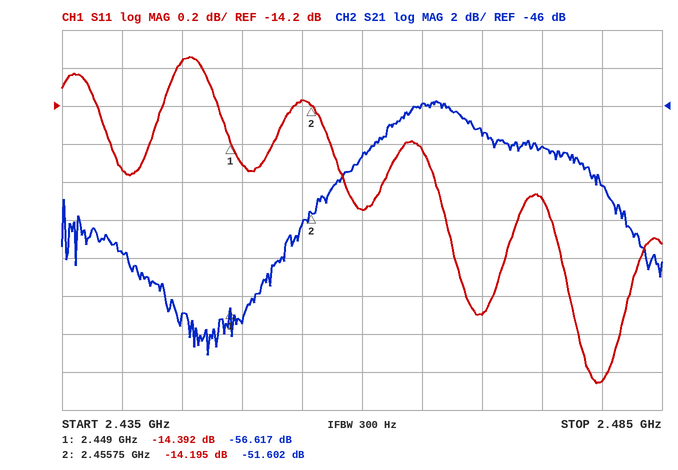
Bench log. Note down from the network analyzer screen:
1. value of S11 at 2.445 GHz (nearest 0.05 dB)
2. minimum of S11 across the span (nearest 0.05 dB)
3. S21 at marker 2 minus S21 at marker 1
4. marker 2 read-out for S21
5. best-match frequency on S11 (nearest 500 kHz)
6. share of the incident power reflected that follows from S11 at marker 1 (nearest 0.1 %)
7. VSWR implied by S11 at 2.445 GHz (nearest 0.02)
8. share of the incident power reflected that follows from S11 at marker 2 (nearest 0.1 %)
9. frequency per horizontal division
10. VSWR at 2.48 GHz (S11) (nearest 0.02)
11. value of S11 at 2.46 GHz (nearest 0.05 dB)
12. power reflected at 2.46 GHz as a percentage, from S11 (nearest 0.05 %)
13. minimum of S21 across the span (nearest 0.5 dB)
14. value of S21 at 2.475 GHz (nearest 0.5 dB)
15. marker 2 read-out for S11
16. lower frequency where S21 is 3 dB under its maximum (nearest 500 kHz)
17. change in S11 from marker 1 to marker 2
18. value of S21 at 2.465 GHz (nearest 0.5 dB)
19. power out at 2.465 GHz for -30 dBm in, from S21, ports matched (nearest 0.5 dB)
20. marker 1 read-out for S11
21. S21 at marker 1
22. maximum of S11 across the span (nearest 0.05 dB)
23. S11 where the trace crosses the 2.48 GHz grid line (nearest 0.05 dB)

-13.95 dB
-15.65 dB
5.015 dB
-51.602 dB
2.4795 GHz
3.6 %
1.50
3.8 %
5 MHz
1.40
-14.75 dB
3.35 %
-59.0 dB
-48.0 dB
-14.195 dB
2.4600 GHz
0.197 dB
-46.0 dB
-76.0 dBm
-14.392 dB
-56.617 dB
-13.95 dB
-15.65 dB
